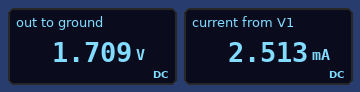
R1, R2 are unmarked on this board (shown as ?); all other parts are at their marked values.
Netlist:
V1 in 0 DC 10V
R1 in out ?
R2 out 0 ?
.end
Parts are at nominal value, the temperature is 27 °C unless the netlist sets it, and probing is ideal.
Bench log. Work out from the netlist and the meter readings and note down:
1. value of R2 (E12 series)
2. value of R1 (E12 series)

680 Ω
3.3 kΩ
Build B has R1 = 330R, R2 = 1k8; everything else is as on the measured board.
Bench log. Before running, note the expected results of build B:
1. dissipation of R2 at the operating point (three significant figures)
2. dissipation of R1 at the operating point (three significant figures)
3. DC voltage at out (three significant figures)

39.7 mW
7.27 mW
8.45 V
